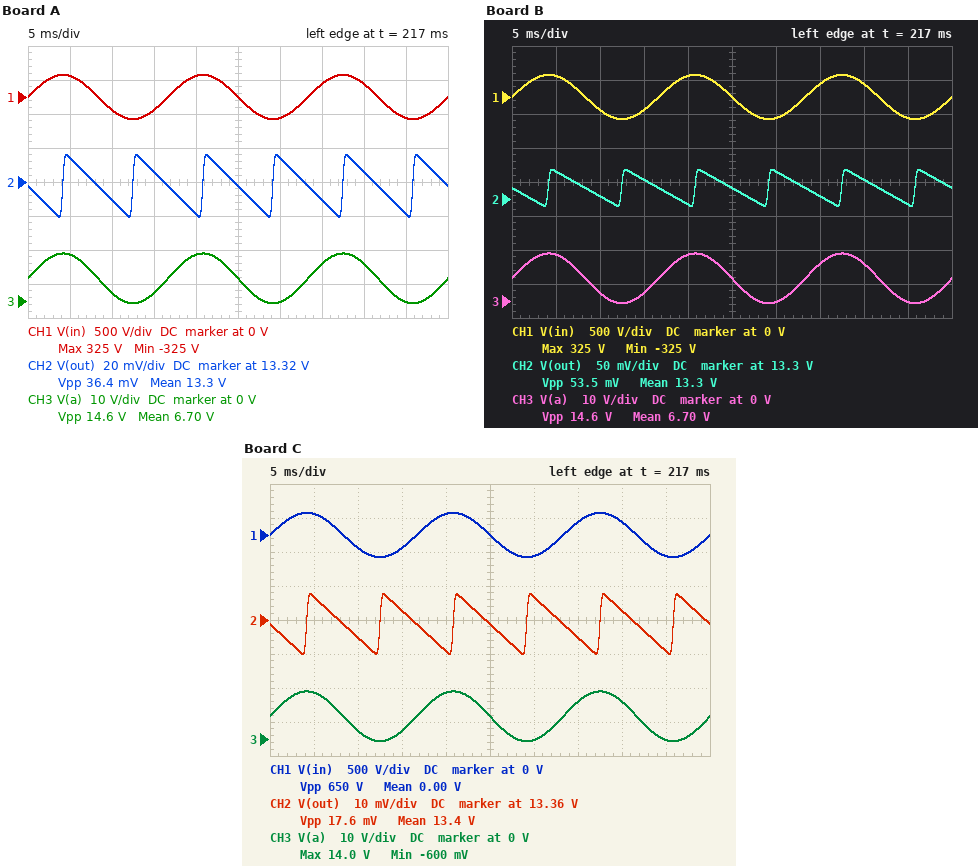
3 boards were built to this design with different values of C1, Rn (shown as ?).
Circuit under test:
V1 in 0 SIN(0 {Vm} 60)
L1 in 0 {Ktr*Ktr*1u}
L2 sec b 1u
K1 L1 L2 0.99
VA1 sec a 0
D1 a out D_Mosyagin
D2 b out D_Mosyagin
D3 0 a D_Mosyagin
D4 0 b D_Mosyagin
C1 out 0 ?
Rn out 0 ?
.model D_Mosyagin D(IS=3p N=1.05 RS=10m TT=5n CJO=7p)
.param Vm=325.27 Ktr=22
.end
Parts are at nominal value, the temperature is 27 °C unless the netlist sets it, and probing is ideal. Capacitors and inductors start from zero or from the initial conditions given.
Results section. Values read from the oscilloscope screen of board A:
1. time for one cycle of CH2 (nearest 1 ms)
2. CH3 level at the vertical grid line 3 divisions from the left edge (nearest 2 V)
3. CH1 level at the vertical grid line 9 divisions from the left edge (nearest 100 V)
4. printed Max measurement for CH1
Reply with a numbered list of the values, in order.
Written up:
1. 8 ms
2. 2 V
3. -300 V
4. 325 V
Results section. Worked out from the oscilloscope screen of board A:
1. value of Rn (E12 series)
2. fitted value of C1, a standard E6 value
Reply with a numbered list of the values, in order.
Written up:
1. 2.7 kΩ
2. 1 mF
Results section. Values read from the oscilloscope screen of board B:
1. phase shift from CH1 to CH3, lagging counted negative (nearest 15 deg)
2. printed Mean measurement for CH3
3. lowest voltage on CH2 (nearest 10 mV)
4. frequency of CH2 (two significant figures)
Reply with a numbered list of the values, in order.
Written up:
1. 0 deg
2. 6.70 V
3. 13.29 V
4. 120 Hz
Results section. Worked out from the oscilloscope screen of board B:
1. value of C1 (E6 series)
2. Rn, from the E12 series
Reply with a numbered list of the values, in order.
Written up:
1. 680 µF
2. 2.7 kΩ
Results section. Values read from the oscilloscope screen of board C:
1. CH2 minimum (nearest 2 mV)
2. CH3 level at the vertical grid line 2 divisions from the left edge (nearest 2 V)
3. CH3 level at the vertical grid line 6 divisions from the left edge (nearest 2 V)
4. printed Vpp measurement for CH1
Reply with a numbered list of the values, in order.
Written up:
1. 13.350 V
2. 2 V
3. 0 V
4. 650 V
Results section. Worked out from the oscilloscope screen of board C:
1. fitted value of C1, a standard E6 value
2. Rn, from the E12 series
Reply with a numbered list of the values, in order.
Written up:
1. 1 mF
2. 5.6 kΩ
